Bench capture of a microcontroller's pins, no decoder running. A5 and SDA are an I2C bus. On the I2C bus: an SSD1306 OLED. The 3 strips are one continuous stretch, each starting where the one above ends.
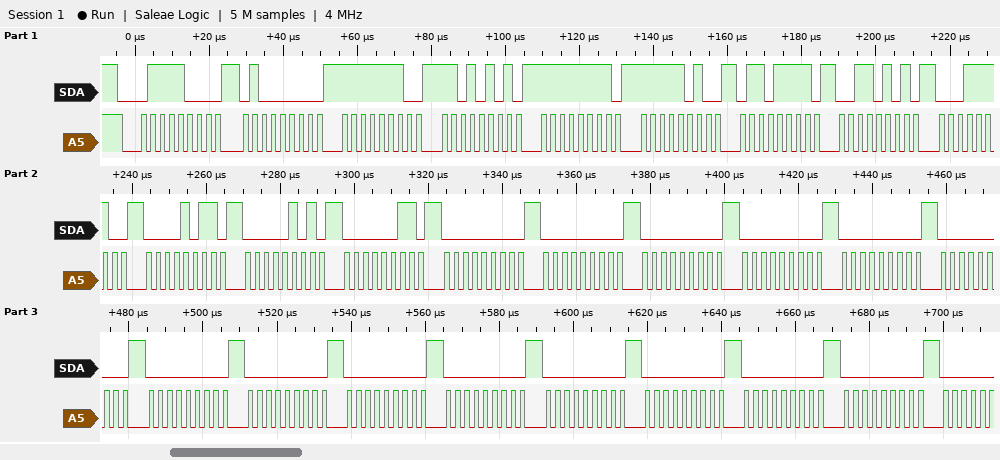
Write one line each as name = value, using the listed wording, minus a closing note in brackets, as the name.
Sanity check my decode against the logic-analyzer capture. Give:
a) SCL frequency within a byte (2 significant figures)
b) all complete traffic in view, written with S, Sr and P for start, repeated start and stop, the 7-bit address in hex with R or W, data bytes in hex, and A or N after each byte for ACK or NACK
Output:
SCL frequency within a byte = 400 kHz
all complete traffic in view, written with S, Sr and P for start, repeated start and stop, the 7-bit address in hex with R or W, data bytes in hex, and A or N after each byte for ACK or NACK = S 3CW A 40 A FE A D5 A FF A FA A 6F A 35 A 1E A 0B A 05 A 03 A 00 A 00 A 00 A 00 A 00 A 00 A 00 A 00 A 00 A 00 A 00 A 00 A 00 A 00 A
